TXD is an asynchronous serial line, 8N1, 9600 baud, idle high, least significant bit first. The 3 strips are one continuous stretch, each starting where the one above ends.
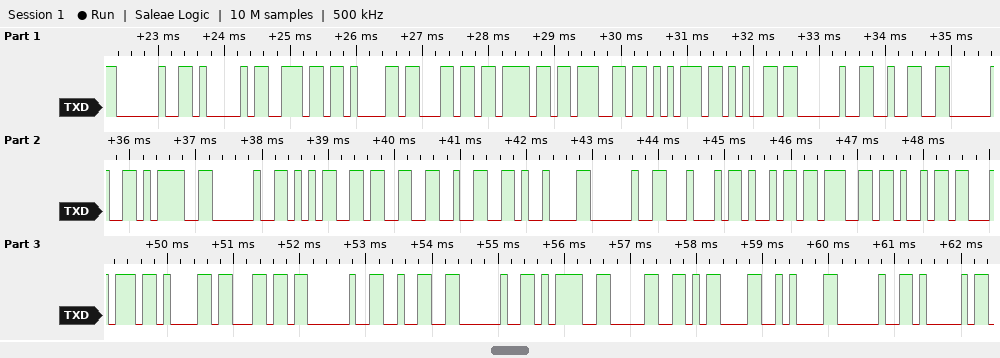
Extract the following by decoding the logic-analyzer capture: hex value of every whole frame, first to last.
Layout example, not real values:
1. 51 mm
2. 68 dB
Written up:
1. 20 41 6E 61 6C 6F 67 75 65 20 32 20 3D 20 35 33 32 09 20 44 69 67 69 74 61 6C 20 32 20 3D 30 0D 0A 20 41
